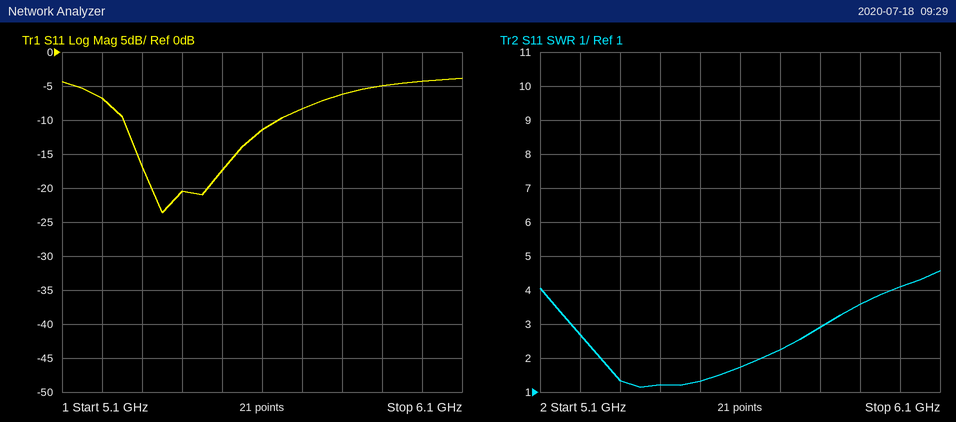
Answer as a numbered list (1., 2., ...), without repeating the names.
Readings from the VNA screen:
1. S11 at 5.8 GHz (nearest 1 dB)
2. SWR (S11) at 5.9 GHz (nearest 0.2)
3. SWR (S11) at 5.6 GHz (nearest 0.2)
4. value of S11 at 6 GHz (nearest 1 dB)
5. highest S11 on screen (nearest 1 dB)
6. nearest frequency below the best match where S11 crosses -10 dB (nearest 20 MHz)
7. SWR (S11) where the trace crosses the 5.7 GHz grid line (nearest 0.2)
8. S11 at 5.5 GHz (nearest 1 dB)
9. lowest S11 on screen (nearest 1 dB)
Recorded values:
1. -6 dB
2. 3.6
3. 1.8
4. -4 dB
5. -4 dB
6. 5.26 GHz
7. 2.2
8. -17 dB
9. -24 dB
